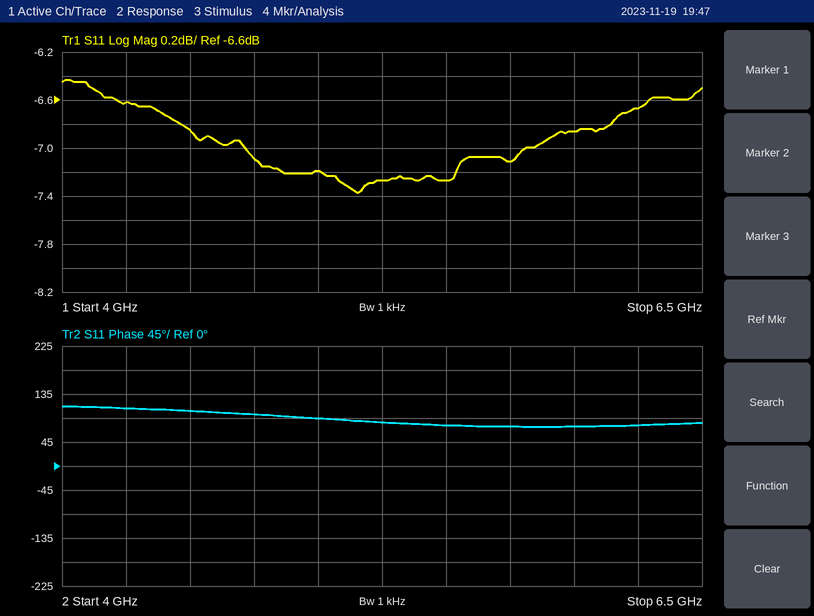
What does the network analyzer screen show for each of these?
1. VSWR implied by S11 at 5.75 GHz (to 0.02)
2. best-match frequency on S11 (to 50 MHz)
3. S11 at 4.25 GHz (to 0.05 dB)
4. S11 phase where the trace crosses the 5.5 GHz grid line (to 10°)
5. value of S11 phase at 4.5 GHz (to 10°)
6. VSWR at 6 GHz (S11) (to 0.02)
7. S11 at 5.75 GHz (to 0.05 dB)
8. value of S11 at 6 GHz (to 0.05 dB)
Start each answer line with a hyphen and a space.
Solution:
- 2.58
- 5.15 GHz
- -6.60 dB
- 80°
- 100°
- 2.66
- -7.10 dB
- -6.85 dB
